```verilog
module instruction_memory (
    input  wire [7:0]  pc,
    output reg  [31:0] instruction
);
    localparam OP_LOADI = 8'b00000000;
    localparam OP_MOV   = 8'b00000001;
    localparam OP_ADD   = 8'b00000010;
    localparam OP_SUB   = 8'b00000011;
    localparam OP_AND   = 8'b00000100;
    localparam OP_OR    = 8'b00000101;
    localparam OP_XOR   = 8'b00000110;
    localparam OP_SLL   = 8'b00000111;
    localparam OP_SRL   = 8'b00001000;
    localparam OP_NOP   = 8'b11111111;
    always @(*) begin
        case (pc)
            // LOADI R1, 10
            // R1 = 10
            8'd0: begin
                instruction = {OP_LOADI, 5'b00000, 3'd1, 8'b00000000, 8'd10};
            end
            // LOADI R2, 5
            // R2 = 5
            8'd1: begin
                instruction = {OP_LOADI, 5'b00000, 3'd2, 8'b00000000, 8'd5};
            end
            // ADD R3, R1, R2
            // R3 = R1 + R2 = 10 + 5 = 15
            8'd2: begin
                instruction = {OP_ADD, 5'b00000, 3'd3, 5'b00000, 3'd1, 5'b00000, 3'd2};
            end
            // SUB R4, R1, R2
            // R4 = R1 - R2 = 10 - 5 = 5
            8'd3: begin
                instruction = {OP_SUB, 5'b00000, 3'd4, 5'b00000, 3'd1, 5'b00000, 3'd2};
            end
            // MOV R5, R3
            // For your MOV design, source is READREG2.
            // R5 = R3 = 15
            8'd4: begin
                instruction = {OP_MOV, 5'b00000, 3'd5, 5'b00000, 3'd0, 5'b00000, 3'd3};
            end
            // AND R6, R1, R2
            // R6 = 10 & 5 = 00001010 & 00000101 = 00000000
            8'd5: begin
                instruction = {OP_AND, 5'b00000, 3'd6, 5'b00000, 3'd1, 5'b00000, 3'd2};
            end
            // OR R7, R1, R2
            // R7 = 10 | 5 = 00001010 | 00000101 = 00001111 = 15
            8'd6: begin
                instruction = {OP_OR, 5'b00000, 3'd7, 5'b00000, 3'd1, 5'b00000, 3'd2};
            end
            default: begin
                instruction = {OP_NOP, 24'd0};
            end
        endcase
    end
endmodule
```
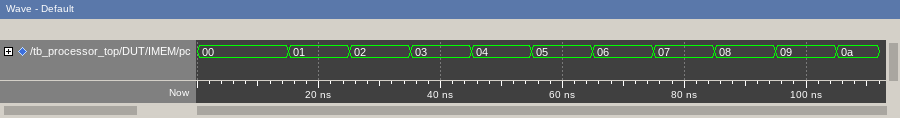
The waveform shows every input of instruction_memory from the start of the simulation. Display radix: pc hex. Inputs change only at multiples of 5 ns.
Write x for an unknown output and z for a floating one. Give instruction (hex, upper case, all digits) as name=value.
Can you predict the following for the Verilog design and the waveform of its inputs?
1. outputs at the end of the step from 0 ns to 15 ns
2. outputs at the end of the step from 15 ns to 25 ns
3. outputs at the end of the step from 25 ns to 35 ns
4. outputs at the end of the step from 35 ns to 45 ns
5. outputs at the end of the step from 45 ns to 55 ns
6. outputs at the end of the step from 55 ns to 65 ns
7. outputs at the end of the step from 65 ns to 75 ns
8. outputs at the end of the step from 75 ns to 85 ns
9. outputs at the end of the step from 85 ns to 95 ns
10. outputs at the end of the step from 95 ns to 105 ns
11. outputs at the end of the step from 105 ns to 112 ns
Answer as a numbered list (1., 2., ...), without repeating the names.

1. instruction=0001000A
2. instruction=00020005
3. instruction=02030102
4. instruction=03040102
5. instruction=01050003
6. instruction=04060102
7. instruction=05070102
8. instruction=FF000000
9. instruction=FF000000
10. instruction=FF000000
11. instruction=FF000000
